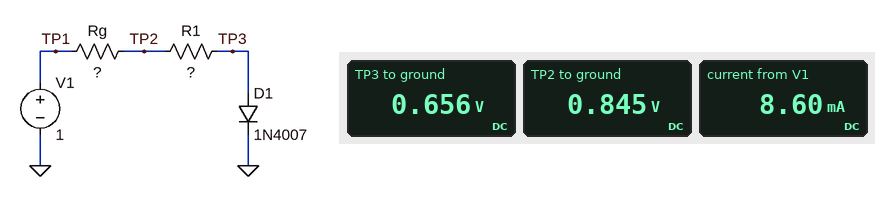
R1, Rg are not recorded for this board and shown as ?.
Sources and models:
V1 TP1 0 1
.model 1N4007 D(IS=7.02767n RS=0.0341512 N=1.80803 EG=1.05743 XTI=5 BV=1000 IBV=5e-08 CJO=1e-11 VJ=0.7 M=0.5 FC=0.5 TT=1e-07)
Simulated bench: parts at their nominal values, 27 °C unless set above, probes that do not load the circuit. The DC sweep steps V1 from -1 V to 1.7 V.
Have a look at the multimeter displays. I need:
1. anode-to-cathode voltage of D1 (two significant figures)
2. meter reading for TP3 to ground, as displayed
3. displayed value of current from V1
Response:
660 mV
0.656 V
8.60 mA
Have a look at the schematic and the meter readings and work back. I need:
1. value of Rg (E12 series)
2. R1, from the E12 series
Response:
18 Ω
22 Ω
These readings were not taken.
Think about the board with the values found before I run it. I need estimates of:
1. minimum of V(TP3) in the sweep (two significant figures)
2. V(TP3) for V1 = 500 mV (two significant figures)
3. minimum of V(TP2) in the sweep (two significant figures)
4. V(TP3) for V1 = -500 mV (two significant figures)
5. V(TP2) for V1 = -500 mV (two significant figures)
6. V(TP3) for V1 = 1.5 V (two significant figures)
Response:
-1.0 V
490 mV
-1.0 V
-500 mV
-500 mV
700 mV
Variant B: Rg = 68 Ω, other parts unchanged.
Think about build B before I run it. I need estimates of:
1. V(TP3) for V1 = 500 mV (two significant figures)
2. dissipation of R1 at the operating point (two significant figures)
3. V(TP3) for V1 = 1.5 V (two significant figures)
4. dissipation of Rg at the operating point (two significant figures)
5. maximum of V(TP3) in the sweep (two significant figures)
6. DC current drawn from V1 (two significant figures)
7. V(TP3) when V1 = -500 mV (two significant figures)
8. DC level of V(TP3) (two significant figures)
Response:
480 mV
390 µW
660 mV
1.2 mW
670 mV
4.2 mA
-500 mV
620 mV
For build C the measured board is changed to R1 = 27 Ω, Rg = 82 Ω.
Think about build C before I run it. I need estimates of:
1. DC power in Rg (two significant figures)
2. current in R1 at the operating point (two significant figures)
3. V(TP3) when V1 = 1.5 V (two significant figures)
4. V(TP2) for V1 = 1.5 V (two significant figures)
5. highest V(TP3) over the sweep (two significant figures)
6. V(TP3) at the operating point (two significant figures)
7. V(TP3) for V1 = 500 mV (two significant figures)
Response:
1.0 mW
3.5 mA
650 mV
860 mV
660 mV
610 mV
480 mV
